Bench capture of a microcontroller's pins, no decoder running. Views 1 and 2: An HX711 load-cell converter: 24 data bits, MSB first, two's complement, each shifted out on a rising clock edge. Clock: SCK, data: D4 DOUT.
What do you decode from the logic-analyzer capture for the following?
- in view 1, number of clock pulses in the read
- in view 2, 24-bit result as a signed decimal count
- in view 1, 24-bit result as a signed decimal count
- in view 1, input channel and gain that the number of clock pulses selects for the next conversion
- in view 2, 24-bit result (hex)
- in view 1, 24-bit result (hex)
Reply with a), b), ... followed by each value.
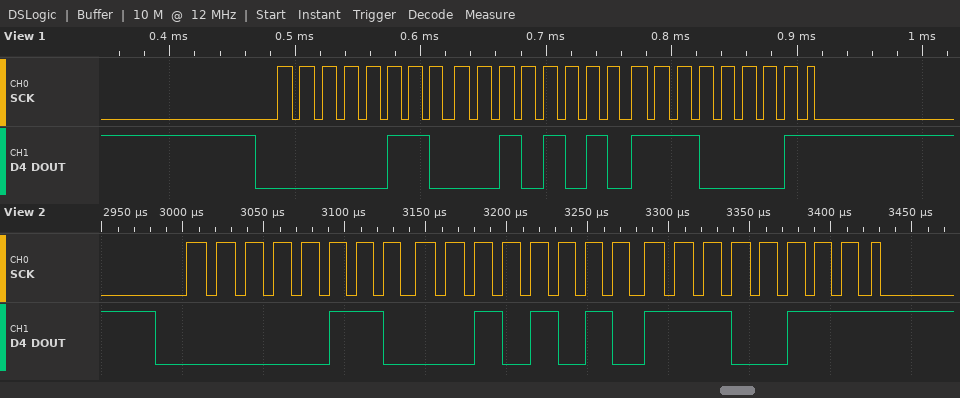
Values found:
a) 25
b) 404199
c) 404193
d) channel A, gain 128
e) 0x062AE7
f) 0x062AE1
